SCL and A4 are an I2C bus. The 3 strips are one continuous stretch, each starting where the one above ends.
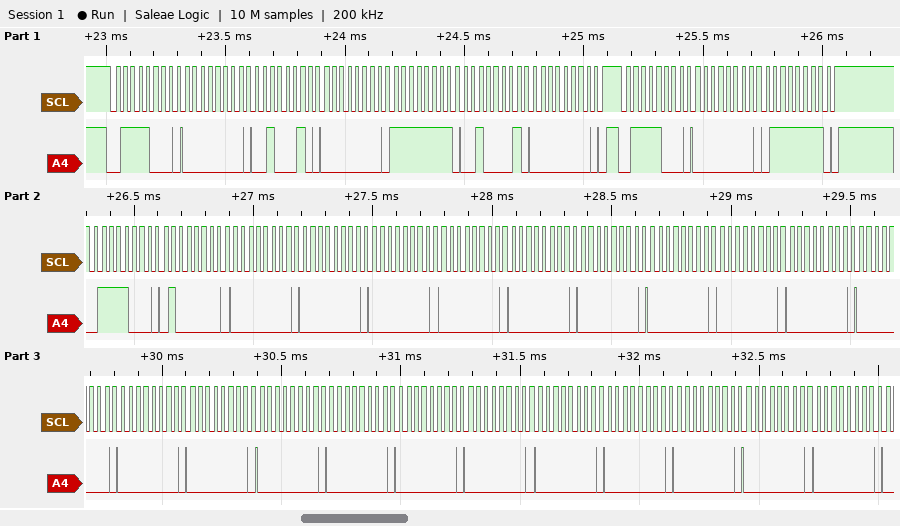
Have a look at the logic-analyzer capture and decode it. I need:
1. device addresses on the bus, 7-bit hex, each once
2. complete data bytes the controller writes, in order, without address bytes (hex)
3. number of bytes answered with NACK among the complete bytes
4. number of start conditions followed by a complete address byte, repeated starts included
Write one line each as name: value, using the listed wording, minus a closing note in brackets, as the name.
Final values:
device addresses on the bus, 7-bit hex, each once: 0x3C
complete data bytes the controller writes, in order, without address bytes: 00 22 00 FF 21 00 00 7F 40 00 00 00 00 00 00 00 00 00 00 00 00 00 00 00 00 00 00 00 00 00
number of bytes answered with NACK among the complete bytes: 0
number of start conditions followed by a complete address byte, repeated starts included: 3
